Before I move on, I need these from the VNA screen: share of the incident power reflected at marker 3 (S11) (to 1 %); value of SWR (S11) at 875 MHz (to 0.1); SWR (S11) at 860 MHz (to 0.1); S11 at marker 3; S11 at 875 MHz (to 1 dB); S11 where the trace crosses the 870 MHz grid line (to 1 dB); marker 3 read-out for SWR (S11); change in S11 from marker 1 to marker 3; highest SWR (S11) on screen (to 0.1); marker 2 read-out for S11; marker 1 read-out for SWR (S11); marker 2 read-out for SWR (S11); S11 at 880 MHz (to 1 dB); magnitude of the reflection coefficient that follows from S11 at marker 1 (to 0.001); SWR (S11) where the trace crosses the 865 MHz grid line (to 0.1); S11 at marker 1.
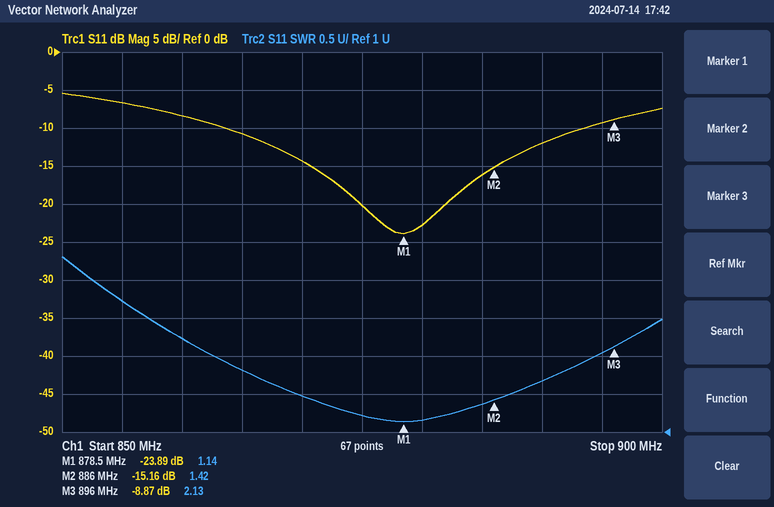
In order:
13 %
1.2
2.2
-8.87 dB
-20 dB
-14 dB
2.13
15.02 dB
3.3
-15.16 dB
1.14
1.42
-23 dB
0.064
1.8
-23.89 dB
